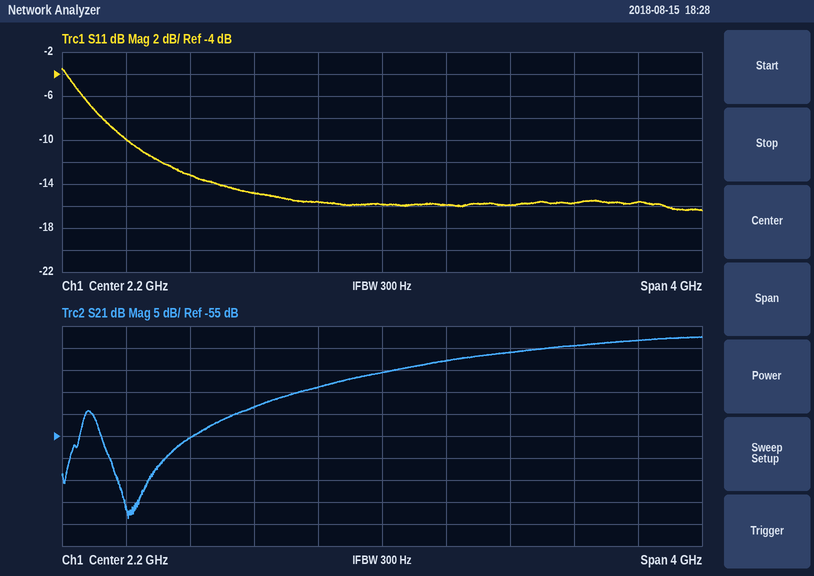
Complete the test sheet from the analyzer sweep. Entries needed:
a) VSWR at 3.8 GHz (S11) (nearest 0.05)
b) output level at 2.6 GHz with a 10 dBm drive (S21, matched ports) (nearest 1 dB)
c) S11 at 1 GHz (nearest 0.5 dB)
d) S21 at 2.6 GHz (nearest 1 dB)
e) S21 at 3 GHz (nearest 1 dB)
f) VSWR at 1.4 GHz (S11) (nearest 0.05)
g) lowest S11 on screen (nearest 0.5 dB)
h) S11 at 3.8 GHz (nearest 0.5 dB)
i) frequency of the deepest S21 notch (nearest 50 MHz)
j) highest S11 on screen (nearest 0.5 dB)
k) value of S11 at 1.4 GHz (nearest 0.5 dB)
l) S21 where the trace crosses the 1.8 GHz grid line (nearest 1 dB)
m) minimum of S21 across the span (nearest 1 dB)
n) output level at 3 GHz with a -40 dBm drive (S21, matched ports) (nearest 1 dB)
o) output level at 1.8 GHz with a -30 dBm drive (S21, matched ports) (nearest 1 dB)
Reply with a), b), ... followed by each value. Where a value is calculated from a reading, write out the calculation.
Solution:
a) |Γ| = 10^(-15.5/20) = 0.1679; VSWR = (1 + 0.1679)/(1 − 0.1679) ≈ 1.40
b) 10 dBm + (-38 dB) = -28 dBm
c) -13.0 dB
d) -38 dB
e) -36 dB
f) |Γ| = 10^(-15/20) = 0.1778; VSWR = (1 + 0.1778)/(1 − 0.1778) ≈ 1.43, so 1.45 to the nearest 0.05
g) -16.5 dB
h) -15.5 dB
i) 600 MHz
j) -3.5 dB
k) -15.0 dB
l) -44 dB
m) -74 dB
n) -40 dBm + (-36 dB) = -76 dBm
o) -30 dBm + (-44 dB) = -74 dBm
